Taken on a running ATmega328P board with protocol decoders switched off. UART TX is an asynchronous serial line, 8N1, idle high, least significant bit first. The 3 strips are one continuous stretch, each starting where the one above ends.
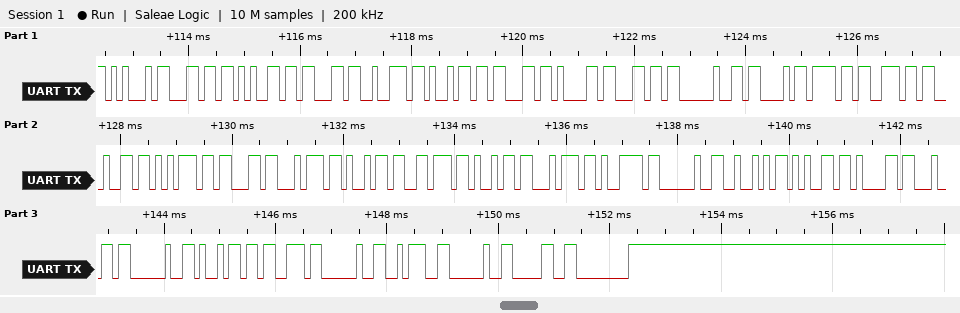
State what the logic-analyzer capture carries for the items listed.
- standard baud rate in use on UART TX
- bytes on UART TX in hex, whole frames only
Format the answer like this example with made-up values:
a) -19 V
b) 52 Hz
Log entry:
a) 9600 baud
b) 45 6C 65 63 72 69 63 61 6C 20 43 6F 6E 64 75 63 74 69 76 69 74 79 20 52 65 61 64 20 69 73 20 3A 20 30 00
